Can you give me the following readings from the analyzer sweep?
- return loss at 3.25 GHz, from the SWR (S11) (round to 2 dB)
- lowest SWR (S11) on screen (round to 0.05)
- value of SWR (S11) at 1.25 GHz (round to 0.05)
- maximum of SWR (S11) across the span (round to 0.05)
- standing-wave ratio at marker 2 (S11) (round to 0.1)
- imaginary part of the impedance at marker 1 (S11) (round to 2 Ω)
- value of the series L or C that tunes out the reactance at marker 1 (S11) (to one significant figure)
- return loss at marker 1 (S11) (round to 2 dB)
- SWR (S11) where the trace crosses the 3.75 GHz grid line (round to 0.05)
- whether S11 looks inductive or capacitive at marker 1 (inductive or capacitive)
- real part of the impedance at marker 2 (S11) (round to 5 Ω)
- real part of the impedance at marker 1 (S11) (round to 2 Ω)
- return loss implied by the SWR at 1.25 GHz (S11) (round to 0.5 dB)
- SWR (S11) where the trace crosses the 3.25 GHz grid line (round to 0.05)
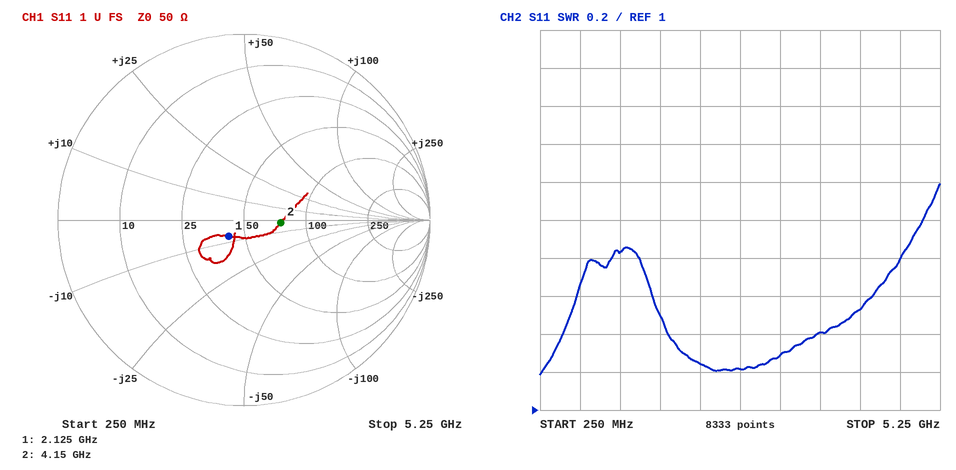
18 dB
1.20
1.85
2.20
1.5
-8 Ω
600 pH
18 dB
1.40
capacitive
75 Ω
42 Ω
10.5 dB
1.30
